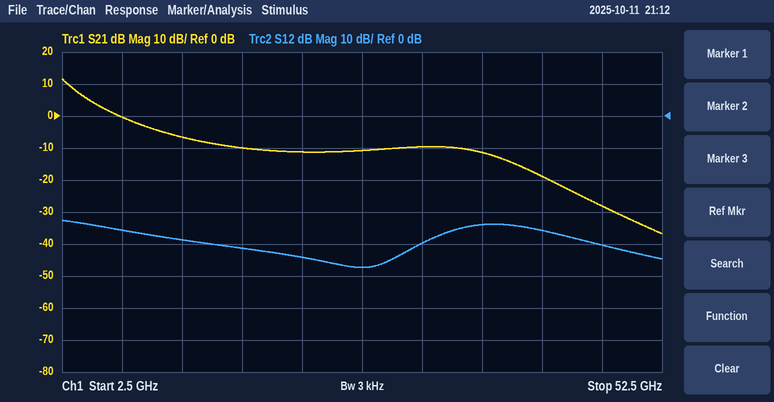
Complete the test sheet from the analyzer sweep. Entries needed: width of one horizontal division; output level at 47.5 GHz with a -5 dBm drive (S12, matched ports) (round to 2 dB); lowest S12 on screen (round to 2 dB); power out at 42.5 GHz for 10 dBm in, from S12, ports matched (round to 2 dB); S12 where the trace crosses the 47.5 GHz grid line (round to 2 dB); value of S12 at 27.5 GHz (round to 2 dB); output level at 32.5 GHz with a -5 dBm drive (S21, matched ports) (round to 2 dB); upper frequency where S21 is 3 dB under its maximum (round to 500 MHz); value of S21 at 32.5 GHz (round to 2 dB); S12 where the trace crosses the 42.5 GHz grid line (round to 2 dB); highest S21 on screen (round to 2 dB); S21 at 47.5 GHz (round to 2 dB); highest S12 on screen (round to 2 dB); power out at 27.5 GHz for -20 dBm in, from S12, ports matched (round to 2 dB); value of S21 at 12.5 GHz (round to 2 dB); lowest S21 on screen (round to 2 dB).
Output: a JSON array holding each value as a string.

["5 GHz", "-46 dBm", "-48 dB", "-26 dBm", "-40 dB", "-48 dB", "-14 dBm", "3.5 GHz", "-10 dB", "-36 dB", "12 dB", "-28 dB", "-32 dB", "-68 dBm", "-6 dB", "-36 dB"]
